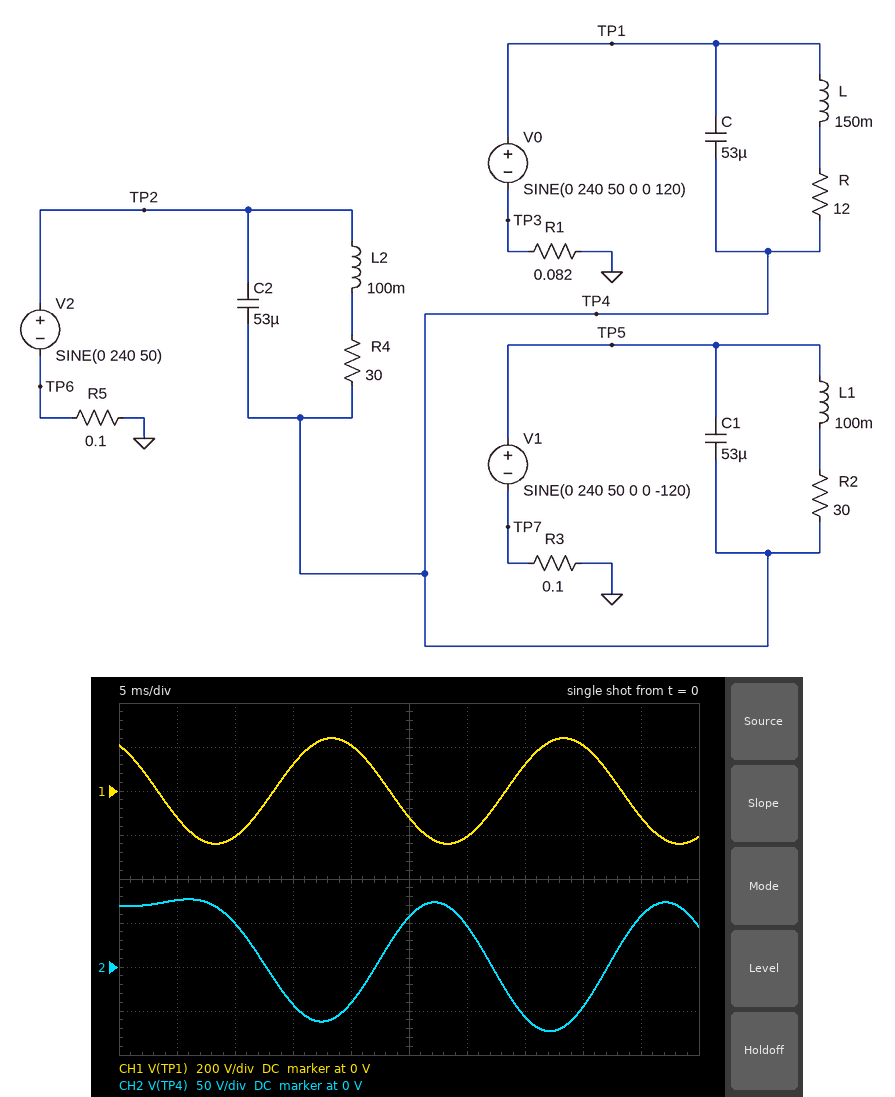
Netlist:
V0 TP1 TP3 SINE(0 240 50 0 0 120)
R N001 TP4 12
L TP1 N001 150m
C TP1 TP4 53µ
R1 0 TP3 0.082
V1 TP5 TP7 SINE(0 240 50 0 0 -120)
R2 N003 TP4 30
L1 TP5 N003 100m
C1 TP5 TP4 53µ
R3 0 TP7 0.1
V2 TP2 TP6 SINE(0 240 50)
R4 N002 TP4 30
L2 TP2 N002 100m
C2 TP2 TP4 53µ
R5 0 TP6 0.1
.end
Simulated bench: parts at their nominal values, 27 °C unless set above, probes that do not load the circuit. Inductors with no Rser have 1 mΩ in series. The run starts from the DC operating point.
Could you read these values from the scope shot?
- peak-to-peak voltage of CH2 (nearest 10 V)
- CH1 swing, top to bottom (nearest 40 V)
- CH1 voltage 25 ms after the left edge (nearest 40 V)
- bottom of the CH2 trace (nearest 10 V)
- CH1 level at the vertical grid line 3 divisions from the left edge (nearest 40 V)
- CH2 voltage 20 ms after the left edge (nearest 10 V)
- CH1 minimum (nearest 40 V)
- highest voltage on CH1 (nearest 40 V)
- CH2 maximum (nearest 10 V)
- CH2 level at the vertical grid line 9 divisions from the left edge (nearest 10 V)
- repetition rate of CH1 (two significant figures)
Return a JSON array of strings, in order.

["150 V", "480 V", "-120 V", "-70 V", "120 V", "-40 V", "-240 V", "240 V", "80 V", "60 V", "50 Hz"]
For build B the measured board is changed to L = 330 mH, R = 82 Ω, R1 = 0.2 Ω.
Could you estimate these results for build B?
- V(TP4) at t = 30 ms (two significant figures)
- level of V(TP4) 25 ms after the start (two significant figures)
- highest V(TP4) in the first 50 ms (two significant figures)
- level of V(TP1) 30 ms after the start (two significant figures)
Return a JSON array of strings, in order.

["84 V", "-49 V", "97 V", "-210 V"]
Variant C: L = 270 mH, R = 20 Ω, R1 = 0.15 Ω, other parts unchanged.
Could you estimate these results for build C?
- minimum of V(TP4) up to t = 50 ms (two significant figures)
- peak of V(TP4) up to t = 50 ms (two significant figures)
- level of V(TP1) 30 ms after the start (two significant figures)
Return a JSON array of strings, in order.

["-98 V", "100 V", "-210 V"]
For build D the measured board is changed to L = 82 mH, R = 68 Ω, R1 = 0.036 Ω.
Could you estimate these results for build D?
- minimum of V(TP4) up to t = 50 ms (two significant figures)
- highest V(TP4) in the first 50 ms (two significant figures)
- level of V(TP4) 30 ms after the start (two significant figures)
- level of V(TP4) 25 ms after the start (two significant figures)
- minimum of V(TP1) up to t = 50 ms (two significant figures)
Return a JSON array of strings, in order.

["-63 V", "63 V", "31 V", "-55 V", "-240 V"]
